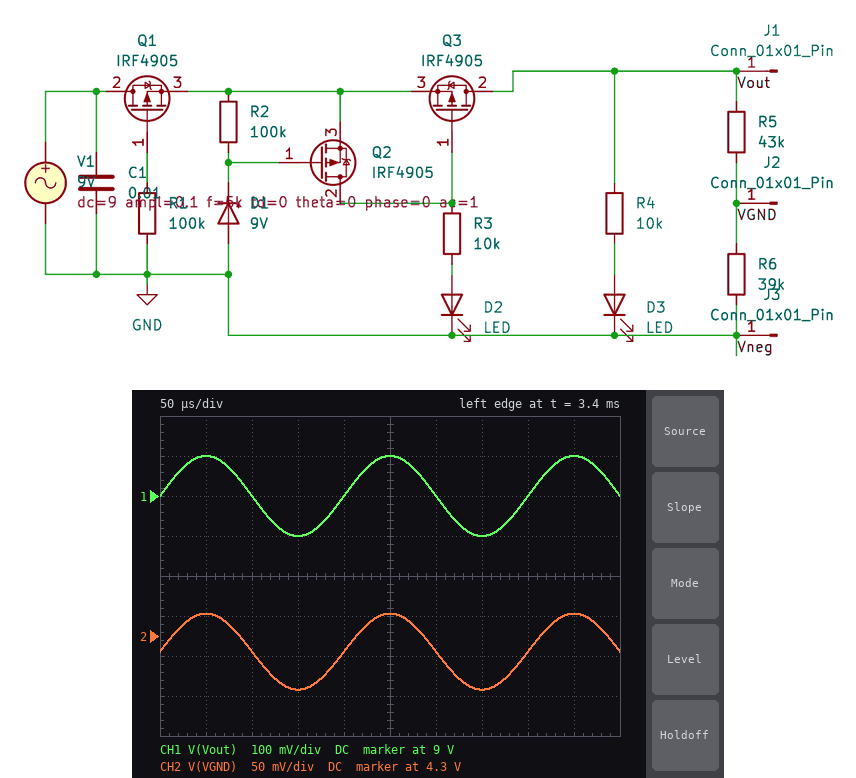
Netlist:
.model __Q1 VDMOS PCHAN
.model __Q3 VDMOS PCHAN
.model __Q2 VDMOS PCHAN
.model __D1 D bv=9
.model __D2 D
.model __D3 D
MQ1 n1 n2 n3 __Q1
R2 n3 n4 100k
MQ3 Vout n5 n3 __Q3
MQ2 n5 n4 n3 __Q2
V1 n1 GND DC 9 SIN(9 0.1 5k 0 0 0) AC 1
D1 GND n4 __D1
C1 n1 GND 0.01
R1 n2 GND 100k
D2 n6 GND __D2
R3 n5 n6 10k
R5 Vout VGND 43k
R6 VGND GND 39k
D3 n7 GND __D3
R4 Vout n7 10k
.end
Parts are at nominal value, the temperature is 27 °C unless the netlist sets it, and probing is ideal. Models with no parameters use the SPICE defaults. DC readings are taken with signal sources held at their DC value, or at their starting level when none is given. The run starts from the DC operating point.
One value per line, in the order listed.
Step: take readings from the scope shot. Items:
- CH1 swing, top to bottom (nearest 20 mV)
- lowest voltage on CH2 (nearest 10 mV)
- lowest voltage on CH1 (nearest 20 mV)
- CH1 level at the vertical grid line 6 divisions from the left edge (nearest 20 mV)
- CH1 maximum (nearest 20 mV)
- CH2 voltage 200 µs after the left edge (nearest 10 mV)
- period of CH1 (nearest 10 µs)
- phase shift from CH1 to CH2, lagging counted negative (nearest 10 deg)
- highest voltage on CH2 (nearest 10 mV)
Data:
200 mV
4.23 V
8.90 V
9.00 V
9.10 V
4.28 V
200 µs
0 deg
4.33 V
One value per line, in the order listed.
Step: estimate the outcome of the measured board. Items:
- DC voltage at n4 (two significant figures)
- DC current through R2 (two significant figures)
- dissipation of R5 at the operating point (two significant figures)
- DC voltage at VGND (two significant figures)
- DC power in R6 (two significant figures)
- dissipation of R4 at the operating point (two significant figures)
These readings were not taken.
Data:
8.8 V
1.7 µA
520 µW
4.3 V
470 µW
7.0 mW
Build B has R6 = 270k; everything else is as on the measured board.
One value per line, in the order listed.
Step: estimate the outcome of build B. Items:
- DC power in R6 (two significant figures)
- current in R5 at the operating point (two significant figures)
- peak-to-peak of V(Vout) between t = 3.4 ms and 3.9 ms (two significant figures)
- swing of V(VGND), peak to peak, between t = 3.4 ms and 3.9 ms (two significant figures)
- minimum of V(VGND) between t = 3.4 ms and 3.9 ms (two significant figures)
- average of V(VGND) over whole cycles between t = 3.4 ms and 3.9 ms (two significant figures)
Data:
220 µW
29 µA
200 mV
170 mV
7.7 V
7.8 V
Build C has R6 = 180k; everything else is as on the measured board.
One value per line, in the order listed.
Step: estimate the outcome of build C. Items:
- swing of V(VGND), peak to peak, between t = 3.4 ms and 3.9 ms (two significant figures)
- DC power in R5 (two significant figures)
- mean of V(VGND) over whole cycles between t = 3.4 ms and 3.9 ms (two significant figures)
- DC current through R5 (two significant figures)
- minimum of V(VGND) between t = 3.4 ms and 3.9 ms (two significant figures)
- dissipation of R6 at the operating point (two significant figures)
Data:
160 mV
70 µW
7.3 V
40 µA
7.2 V
290 µW
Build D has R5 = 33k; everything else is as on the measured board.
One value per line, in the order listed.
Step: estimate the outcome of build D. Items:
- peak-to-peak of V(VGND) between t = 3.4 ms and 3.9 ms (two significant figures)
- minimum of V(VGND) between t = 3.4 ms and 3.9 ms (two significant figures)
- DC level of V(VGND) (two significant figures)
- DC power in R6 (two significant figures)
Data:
110 mV
4.8 V
4.9 V
610 µW
